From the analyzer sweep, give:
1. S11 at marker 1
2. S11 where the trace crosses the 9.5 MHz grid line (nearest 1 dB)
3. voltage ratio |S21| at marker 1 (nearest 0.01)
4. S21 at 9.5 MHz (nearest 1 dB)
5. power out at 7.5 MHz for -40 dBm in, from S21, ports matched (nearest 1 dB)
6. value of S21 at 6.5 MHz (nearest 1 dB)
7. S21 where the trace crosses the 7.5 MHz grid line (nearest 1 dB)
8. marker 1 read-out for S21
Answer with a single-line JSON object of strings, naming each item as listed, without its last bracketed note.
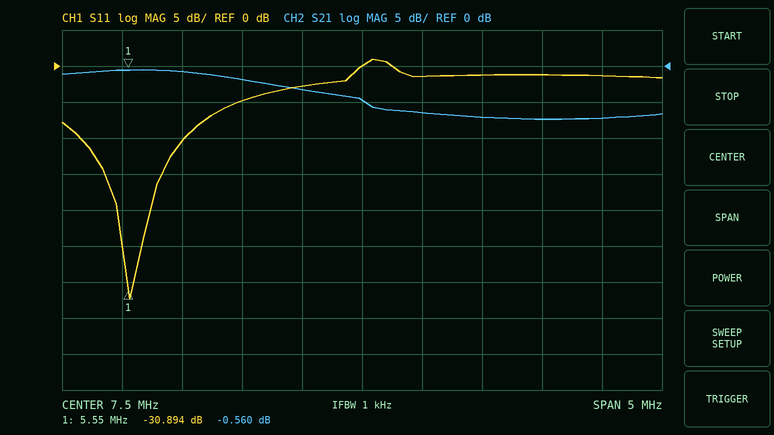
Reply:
{"S11 at marker 1": "-30.894 dB", "S11 where the trace crosses the 9.5 MHz grid line": "-1 dB", "voltage ratio |S21| at marker 1": "0.94", "S21 at 9.5 MHz": "-7 dB", "power out at 7.5 MHz for -40 dBm in, from S21, ports matched": "-45 dBm", "value of S21 at 6.5 MHz": "-2 dB", "S21 where the trace crosses the 7.5 MHz grid line": "-5 dB", "marker 1 read-out for S21": "-0.560 dB"}
